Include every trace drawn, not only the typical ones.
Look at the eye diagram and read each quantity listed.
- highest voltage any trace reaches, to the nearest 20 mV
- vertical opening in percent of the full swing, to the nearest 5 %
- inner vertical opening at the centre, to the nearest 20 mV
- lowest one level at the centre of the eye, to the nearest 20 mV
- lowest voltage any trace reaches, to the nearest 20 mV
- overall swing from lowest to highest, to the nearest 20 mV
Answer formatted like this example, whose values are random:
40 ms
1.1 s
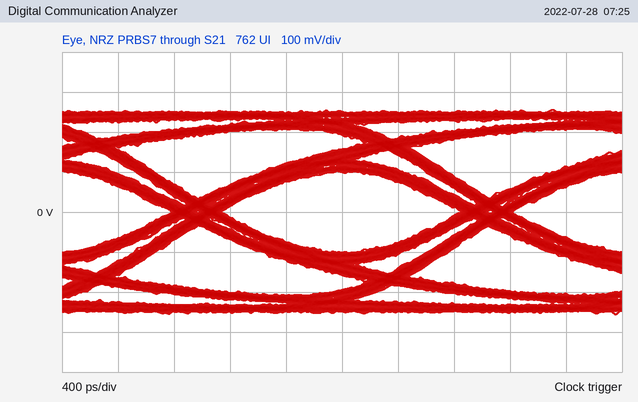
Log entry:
260 mV
40 %
200 mV
100 mV
-260 mV
520 mV
